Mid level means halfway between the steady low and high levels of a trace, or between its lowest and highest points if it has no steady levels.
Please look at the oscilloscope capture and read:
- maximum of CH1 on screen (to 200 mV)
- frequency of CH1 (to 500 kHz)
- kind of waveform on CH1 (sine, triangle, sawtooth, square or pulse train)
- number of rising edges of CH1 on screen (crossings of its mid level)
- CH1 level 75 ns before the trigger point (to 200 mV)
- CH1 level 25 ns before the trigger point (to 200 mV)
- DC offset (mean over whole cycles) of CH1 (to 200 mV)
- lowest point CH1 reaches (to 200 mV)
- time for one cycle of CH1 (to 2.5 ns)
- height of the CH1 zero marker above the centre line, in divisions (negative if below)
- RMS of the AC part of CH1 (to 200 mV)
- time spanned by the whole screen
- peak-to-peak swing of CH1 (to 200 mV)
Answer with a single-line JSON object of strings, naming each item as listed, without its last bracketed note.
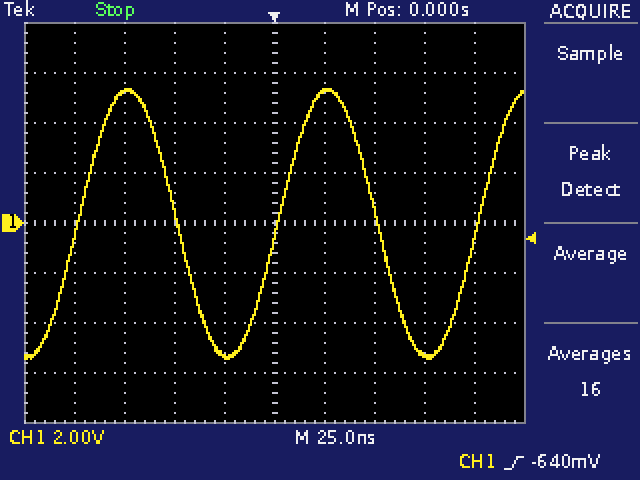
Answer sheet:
{"maximum of CH1 on screen": "5.4 V", "frequency of CH1": "10.0 MHz", "kind of waveform on CH1": "sine", "number of rising edges of CH1 on screen": "3", "CH1 level 75 ns before the trigger point": "5.2 V", "CH1 level 25 ns before the trigger point": "-5.2 V", "DC offset (mean over whole cycles) of CH1": "0.0 V", "lowest point CH1 reaches": "-5.4 V", "time for one cycle of CH1": "100.0 ns", "height of the CH1 zero marker above the centre line, in divisions": "0.0 div", "RMS of the AC part of CH1": "3.8 V", "time spanned by the whole screen": "250 ns", "peak-to-peak swing of CH1": "10.8 V"}
